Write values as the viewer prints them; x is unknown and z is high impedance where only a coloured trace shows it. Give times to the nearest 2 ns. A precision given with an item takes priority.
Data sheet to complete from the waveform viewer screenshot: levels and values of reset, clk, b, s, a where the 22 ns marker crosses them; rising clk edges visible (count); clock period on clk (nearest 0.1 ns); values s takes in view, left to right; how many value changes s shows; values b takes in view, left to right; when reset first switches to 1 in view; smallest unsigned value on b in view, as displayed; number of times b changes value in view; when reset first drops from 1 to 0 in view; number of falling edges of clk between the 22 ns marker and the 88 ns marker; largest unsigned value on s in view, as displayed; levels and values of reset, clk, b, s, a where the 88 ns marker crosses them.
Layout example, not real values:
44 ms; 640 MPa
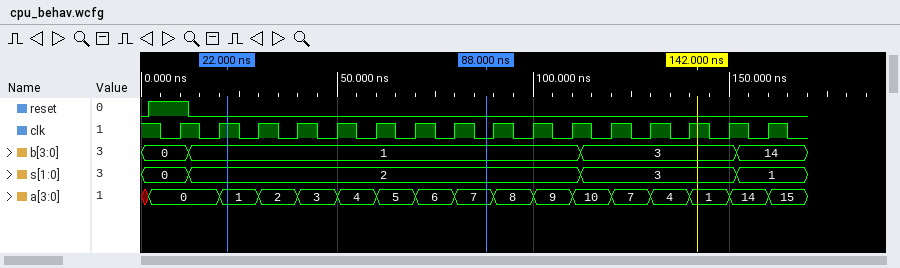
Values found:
reset=0, clk=1, b=1, s=2, a=1; 16; 10 ns; 0, 2, 3, 1; 3; 0, 1, 3, 14; 2 ns; 0; 3; 12 ns; 7; 3; reset=0, clk=0, b=1, s=2, a=7
